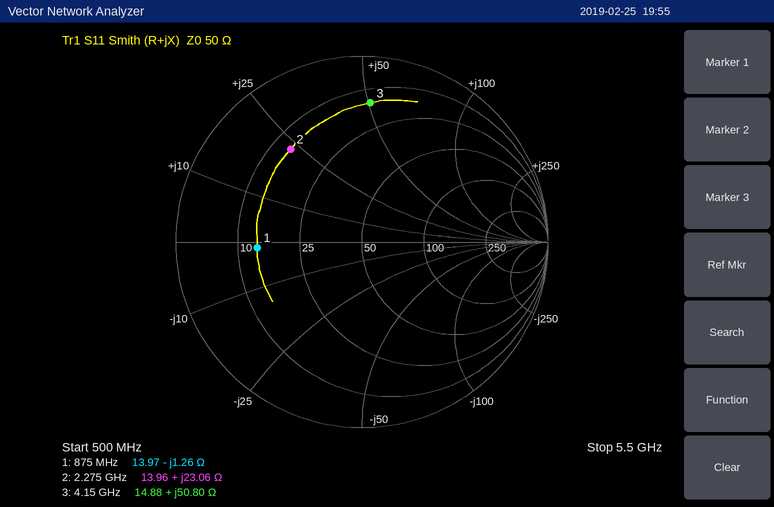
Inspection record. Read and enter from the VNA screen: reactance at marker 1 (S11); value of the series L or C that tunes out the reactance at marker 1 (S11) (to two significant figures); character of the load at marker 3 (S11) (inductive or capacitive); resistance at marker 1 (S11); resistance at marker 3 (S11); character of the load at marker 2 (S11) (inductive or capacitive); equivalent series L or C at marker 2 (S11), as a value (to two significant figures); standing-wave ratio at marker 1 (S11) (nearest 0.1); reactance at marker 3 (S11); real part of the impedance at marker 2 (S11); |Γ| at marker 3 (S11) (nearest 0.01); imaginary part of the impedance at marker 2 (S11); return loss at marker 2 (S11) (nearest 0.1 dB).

-1.26 Ω
230 pH
inductive
13.97 Ω
14.88 Ω
inductive
1.6 nH
3.6
+50.80 Ω
13.96 Ω
0.75
+23.06 Ω
4.0 dB
